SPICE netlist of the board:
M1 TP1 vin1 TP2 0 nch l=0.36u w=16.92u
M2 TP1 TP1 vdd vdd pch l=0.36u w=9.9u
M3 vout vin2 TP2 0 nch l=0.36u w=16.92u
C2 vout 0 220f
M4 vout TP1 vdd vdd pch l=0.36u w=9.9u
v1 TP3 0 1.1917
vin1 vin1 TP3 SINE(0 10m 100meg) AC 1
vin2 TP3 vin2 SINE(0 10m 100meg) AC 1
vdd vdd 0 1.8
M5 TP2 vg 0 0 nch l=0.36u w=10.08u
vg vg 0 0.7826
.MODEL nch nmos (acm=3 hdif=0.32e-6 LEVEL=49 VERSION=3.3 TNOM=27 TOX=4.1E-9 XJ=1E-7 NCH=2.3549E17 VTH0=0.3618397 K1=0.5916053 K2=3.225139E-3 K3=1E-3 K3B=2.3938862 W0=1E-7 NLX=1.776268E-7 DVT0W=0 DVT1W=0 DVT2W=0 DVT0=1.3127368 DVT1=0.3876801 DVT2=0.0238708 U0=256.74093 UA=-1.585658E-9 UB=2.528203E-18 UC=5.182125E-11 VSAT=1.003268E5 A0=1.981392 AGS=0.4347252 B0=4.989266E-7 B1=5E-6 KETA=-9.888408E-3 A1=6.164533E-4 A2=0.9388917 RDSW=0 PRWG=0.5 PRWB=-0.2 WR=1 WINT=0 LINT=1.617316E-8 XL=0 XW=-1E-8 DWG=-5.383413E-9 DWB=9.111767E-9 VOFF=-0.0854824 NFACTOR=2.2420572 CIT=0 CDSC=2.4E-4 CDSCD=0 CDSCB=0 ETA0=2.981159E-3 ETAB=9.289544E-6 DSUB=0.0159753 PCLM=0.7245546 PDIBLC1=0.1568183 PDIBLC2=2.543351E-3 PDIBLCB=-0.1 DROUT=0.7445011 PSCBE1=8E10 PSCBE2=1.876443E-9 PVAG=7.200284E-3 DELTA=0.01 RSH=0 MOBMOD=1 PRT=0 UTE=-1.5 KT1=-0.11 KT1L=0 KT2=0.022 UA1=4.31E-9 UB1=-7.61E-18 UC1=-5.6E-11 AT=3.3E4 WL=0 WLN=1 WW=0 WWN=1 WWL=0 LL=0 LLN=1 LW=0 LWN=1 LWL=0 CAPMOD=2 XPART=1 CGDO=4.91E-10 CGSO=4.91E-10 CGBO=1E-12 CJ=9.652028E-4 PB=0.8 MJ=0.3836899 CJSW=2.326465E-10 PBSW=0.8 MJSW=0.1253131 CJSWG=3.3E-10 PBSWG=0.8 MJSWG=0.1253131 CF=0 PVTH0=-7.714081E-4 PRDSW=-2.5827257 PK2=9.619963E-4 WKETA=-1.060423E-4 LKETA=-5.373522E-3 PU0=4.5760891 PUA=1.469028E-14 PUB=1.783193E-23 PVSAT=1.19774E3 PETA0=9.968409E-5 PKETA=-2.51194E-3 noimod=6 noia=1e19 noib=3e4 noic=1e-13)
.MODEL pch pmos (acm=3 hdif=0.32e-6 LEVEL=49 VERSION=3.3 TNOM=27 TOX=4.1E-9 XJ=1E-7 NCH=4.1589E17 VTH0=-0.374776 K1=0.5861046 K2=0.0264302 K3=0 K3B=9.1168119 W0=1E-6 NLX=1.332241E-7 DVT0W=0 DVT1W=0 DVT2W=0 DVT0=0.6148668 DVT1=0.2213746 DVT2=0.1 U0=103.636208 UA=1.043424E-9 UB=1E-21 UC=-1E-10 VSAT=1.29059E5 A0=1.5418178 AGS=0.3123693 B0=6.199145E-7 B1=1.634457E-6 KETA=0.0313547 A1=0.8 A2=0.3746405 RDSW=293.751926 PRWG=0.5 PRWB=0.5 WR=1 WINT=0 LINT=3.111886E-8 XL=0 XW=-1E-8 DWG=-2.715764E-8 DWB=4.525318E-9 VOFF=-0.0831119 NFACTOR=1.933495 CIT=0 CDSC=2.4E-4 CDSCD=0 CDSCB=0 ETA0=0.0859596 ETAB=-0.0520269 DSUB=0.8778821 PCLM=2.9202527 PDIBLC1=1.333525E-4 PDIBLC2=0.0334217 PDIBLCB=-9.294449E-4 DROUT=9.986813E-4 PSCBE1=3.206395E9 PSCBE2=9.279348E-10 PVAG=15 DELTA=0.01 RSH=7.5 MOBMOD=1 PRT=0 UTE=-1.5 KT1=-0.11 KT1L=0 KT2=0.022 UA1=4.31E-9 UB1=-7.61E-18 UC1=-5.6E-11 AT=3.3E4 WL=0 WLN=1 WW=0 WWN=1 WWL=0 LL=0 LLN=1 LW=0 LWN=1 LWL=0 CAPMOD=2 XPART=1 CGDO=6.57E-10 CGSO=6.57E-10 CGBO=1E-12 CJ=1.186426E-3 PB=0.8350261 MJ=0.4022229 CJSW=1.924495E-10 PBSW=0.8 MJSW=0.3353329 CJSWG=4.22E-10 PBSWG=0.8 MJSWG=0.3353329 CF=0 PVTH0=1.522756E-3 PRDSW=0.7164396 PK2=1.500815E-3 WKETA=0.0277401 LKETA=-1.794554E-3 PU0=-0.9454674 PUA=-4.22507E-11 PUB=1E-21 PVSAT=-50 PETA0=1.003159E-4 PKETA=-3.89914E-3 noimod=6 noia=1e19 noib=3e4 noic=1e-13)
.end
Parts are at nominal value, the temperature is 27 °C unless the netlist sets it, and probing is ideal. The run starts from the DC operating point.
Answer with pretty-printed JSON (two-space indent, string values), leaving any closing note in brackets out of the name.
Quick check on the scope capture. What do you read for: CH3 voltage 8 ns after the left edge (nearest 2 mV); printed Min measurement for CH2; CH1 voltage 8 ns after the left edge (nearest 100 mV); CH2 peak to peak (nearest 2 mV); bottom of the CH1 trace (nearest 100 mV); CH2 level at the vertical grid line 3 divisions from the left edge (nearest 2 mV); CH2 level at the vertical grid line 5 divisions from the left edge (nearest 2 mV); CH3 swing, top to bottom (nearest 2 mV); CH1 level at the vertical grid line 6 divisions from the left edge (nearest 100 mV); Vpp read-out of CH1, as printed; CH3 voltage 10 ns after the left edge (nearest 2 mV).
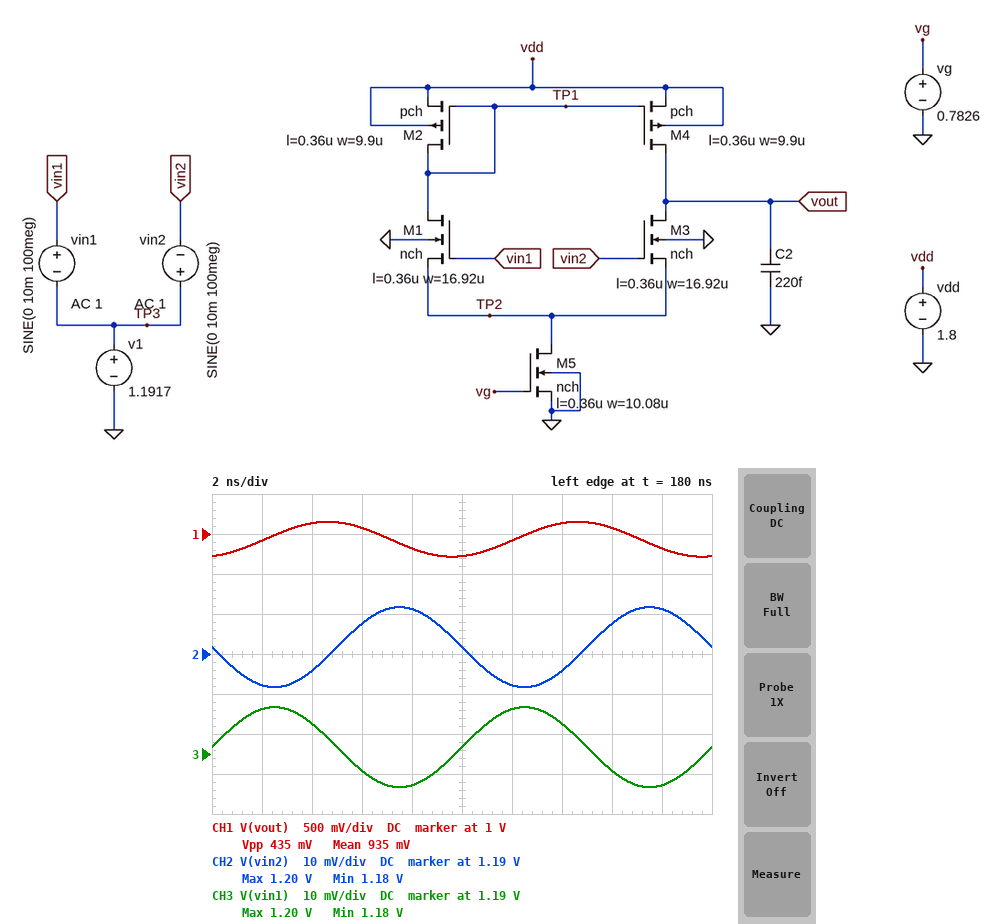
{
  "CH3 voltage 8 ns after the left edge": "1.182 V",
  "printed Min measurement for CH2": "1.18 V",
  "CH1 voltage 8 ns after the left edge": "800 mV",
  "CH2 peak to peak": "20 mV",
  "bottom of the CH1 trace": "700 mV",
  "CH2 level at the vertical grid line 3 divisions from the left edge": "1.198 V",
  "CH2 level at the vertical grid line 5 divisions from the left edge": "1.192 V",
  "CH3 swing, top to bottom": "20 mV",
  "CH1 level at the vertical grid line 6 divisions from the left edge": "900 mV",
  "Vpp read-out of CH1, as printed": "435 mV",
  "CH3 voltage 10 ns after the left edge": "1.192 V"
}
